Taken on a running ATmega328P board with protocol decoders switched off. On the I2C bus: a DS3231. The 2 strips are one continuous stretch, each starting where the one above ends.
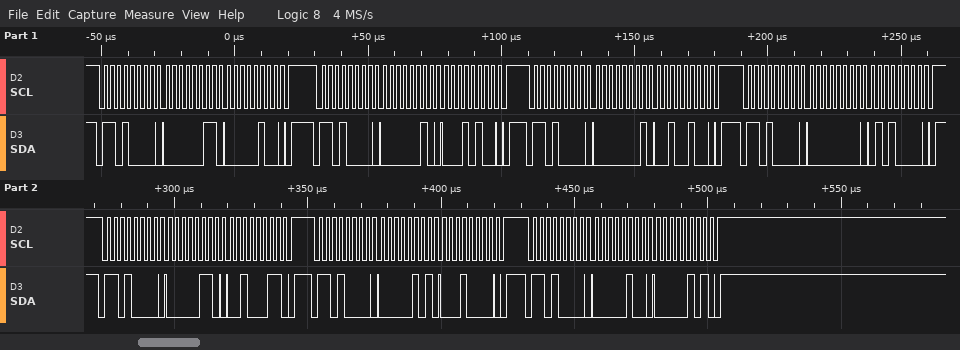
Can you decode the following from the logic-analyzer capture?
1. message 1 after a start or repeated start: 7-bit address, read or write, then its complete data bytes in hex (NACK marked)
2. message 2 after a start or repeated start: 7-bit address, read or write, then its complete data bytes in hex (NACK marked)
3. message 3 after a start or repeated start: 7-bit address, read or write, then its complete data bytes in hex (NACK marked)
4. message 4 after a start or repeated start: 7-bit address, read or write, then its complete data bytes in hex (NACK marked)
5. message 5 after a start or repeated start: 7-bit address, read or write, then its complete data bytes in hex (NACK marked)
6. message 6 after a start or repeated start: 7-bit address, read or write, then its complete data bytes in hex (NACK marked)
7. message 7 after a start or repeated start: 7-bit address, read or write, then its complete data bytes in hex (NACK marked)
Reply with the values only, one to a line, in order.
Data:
0x68 write: 03 04
0x68 write: 02 14
0x68 write: 01 24
0x68 write: 00 50
0x68 write: 06 23
0x68 write: 05 10
0x68 write: 04 05
